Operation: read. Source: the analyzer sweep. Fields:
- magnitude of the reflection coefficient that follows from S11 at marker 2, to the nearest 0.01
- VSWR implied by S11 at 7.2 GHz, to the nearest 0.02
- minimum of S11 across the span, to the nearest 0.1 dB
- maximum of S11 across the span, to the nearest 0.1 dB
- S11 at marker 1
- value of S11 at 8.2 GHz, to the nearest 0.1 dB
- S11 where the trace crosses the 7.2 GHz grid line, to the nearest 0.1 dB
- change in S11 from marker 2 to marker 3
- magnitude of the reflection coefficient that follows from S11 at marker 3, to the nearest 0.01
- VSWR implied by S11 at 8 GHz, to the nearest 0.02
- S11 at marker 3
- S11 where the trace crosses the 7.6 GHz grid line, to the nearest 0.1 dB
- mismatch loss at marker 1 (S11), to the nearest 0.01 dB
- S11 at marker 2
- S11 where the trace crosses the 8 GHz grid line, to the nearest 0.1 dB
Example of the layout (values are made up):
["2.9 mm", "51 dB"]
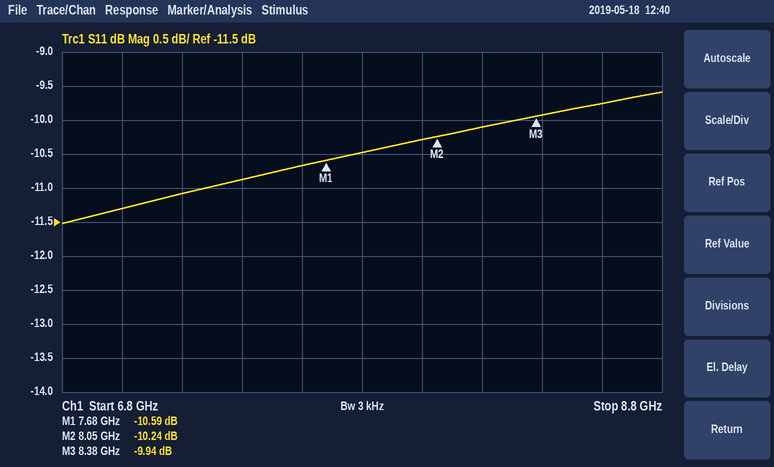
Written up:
["0.31", "1.78", "-11.5 dB", "-9.6 dB", "-10.59 dB", "-10.1 dB", "-11.1 dB", "0.30 dB", "0.32", "1.88", "-9.94 dB", "-10.7 dB", "0.40 dB", "-10.24 dB", "-10.3 dB"]
